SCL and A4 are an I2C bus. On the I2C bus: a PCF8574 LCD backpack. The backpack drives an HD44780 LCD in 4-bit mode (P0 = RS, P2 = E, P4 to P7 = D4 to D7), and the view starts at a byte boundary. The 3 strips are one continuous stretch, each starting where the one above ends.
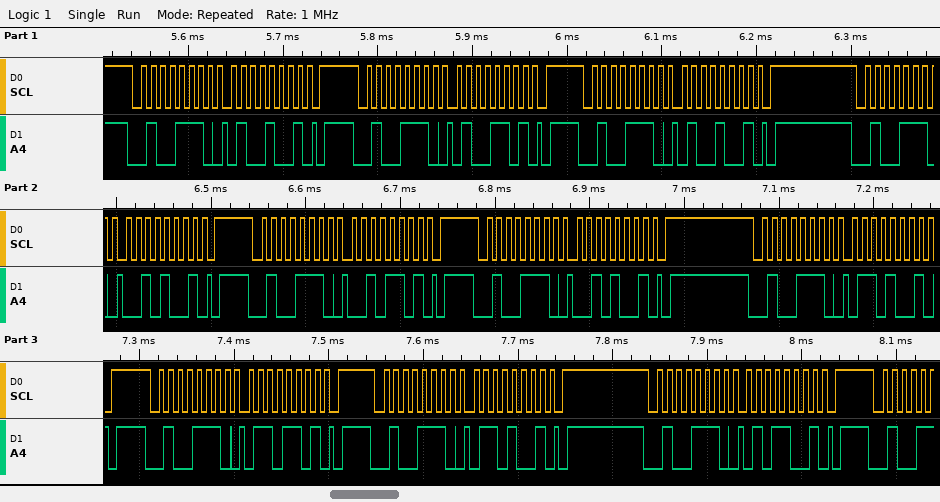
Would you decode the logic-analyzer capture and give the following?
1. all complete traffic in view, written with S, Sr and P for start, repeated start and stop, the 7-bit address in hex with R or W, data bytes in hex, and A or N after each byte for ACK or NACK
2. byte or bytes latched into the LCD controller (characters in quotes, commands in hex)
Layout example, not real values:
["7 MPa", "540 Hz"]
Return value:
["S 27W A 49 A P S 27W A 4D A P S 27W A 49 A P S 27W A 29 A P S 27W A 2D A P S 27W A 29 A P S 27W A 69 A P S 27W A 6D A P S 27W A 69 A P S 27W A 59 A P", "'B'"]
